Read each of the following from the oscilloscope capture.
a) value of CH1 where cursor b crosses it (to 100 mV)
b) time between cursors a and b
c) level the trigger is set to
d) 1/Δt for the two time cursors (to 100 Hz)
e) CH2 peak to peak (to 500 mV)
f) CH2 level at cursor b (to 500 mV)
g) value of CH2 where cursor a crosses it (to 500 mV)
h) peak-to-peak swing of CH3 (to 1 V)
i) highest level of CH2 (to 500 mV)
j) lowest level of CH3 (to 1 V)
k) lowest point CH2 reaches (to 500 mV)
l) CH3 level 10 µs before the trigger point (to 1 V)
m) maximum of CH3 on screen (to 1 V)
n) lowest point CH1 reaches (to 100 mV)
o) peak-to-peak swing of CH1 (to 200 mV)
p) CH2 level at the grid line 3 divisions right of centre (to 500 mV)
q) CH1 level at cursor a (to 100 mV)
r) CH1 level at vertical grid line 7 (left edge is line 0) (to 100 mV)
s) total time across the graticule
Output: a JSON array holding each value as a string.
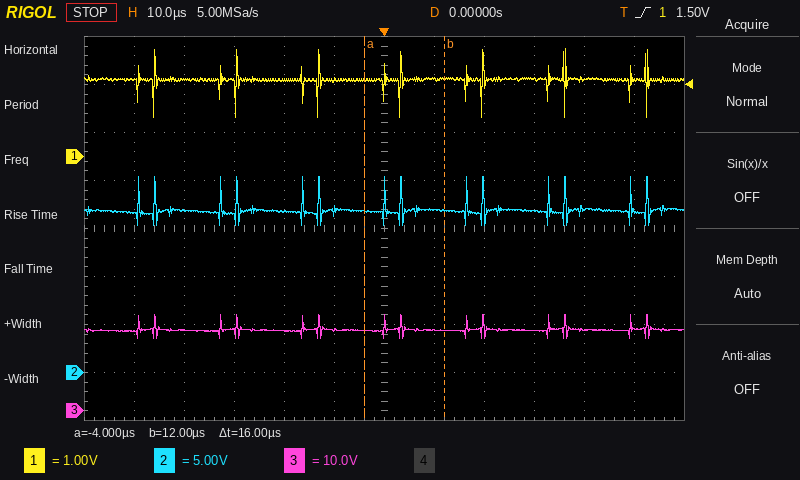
["1.6 V", "16 µs", "1.50 V", "62.5 kHz", "5.0 V", "17.0 V", "17.0 V", "5 V", "20.5 V", "15 V", "15.5 V", "17 V", "20 V", "800 mV", "1.4 V", "17.0 V", "1.6 V", "1.6 V", "120 µs"]
